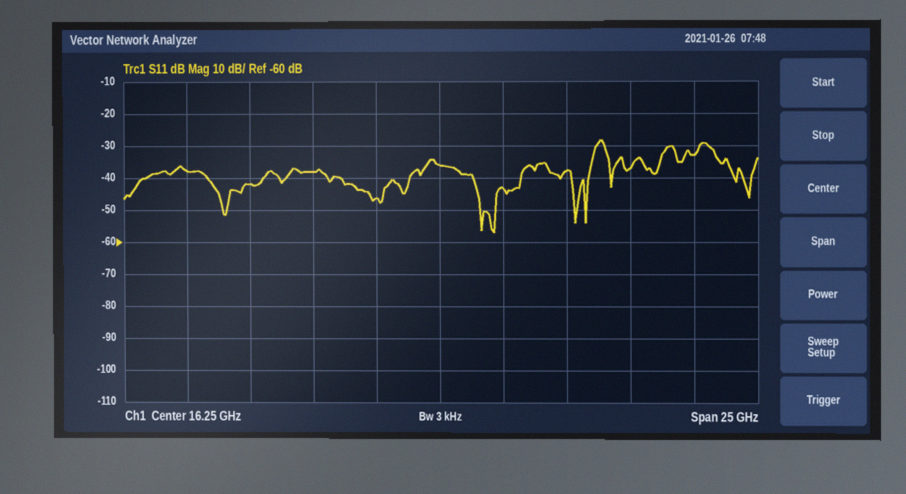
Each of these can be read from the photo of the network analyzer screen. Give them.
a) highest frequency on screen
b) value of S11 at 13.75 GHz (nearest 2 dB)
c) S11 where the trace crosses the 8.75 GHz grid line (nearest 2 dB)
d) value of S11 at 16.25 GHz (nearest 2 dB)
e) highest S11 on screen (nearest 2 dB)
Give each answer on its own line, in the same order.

28.75 GHz
-46 dB
-42 dB
-36 dB
-28 dB
